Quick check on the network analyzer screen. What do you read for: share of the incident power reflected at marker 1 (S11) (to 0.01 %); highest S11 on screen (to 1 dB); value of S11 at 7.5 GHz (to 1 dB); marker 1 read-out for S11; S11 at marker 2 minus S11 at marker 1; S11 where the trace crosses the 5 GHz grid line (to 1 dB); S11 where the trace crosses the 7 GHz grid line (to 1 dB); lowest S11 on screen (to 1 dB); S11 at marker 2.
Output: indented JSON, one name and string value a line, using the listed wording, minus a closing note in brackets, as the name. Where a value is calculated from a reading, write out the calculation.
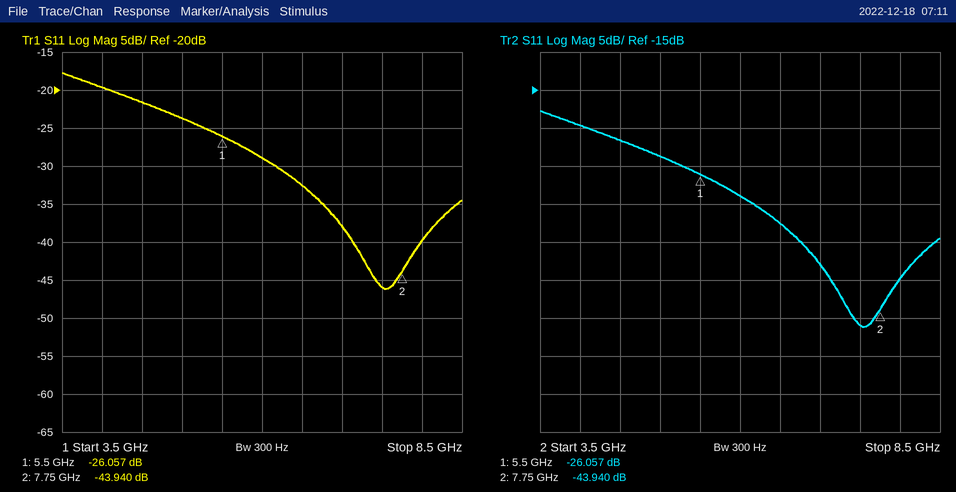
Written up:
{
  "share of the incident power reflected at marker 1 (S11)": "10^(-26.057/10) ≈ 0.25 %",
  "highest S11 on screen": "-18 dB",
  "value of S11 at 7.5 GHz": "-46 dB",
  "marker 1 read-out for S11": "-26.057 dB",
  "S11 at marker 2 minus S11 at marker 1": "-43.94 − (-26.057) = -17.883 dB",
  "S11 where the trace crosses the 5 GHz grid line": "-24 dB",
  "S11 where the trace crosses the 7 GHz grid line": "-38 dB",
  "lowest S11 on screen": "-46 dB",
  "S11 at marker 2": "-43.940 dB"
}
